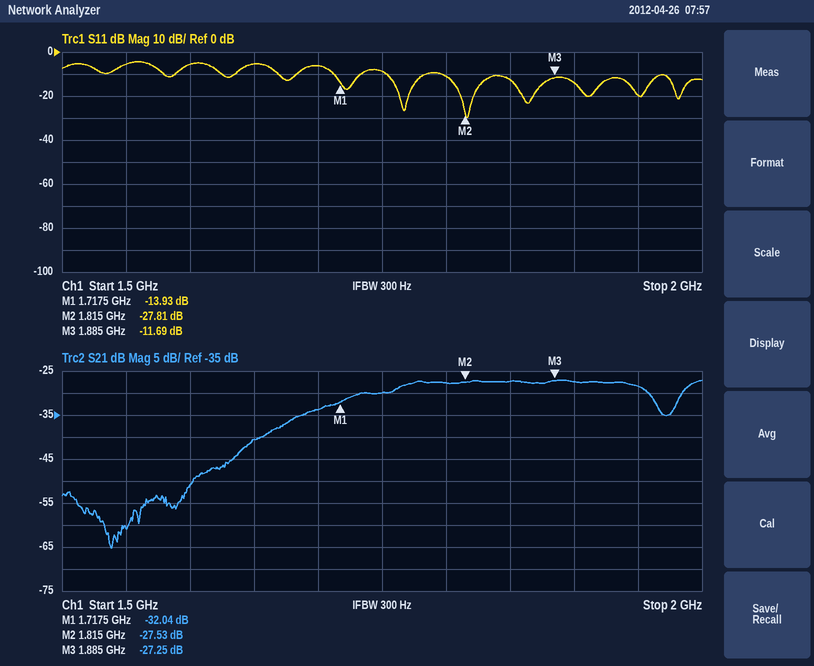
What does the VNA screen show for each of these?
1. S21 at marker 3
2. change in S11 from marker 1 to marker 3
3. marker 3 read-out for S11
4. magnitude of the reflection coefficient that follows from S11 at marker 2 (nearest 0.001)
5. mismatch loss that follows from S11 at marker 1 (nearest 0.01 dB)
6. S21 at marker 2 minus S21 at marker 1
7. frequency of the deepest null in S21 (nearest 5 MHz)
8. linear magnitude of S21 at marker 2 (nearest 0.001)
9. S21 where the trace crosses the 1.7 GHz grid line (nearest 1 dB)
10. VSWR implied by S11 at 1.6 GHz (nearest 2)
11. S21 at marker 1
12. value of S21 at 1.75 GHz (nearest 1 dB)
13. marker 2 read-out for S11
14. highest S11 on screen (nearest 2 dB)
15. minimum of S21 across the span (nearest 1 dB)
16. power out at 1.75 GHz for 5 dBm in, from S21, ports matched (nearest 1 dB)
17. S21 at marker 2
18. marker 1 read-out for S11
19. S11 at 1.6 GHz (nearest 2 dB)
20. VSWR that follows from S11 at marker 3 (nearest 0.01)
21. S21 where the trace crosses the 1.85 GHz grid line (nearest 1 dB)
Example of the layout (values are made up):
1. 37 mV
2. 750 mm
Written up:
1. -27.25 dB
2. 2.24 dB
3. -11.69 dB
4. 0.041
5. 0.18 dB
6. 4.51 dB
7. 1.540 GHz
8. 0.042
9. -34 dB
10. 4
11. -32.04 dB
12. -30 dB
13. -27.81 dB
14. -4 dB
15. -65 dB
16. -25 dBm
17. -27.53 dB
18. -13.93 dB
19. -6 dB
20. 1.70
21. -27 dB
